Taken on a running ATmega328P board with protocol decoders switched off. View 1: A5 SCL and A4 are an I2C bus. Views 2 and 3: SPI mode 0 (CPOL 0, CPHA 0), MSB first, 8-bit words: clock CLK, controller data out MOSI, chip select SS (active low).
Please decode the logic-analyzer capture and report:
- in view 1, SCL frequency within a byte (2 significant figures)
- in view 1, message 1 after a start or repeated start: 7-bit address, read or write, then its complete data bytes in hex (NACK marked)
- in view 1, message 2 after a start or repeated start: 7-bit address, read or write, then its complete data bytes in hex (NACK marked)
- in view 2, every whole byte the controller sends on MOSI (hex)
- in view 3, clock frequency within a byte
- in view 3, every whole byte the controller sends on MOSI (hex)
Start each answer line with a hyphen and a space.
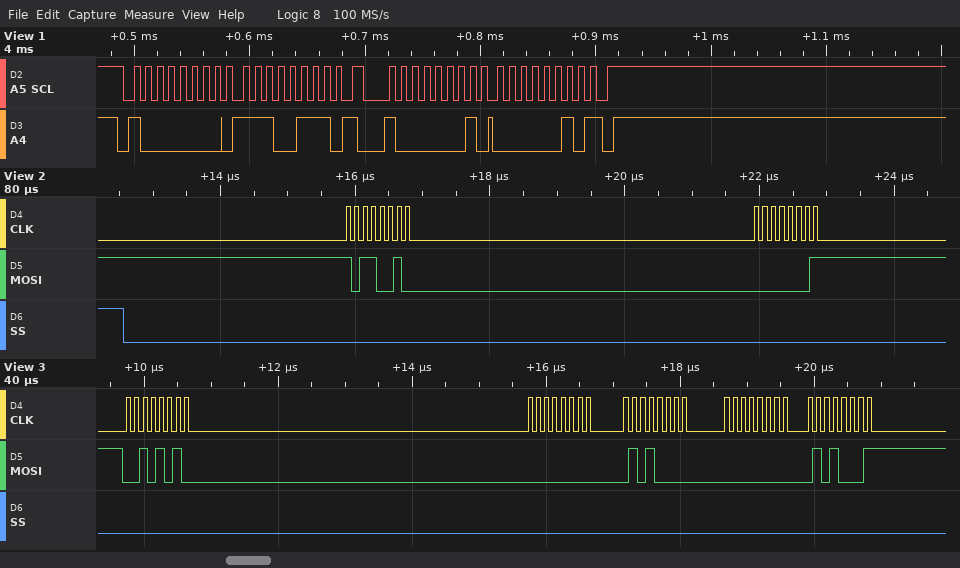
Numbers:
- 100 kHz
- 0x40 write: E7
- 0x40 read: 02 NACK
- B2 01
- 8 MHz
- 2A 00 50 00 51
